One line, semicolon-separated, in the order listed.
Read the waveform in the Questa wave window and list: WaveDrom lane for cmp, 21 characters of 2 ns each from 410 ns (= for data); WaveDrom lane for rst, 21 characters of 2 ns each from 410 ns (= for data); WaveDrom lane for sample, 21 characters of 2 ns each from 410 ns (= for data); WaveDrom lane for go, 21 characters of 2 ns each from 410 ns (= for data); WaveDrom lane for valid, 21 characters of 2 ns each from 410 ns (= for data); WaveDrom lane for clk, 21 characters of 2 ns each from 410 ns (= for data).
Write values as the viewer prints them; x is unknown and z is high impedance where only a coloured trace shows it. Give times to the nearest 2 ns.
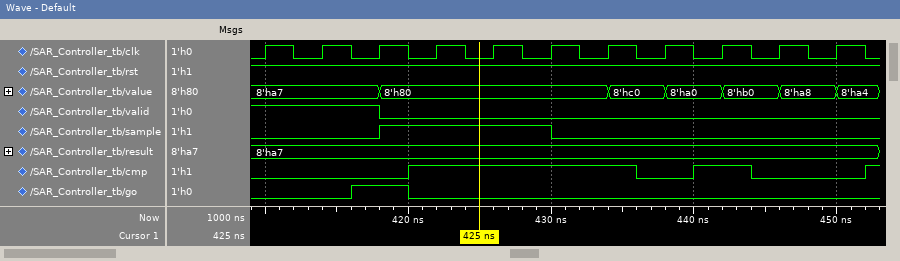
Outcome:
{name: 'cmp', wave: '0....1.......0.1.0...'}; {name: 'rst', wave: '1....................'}; {name: 'sample', wave: '0...1.....0..........'}; {name: 'go', wave: '0..1.0...............'}; {name: 'valid', wave: '1...0................'}; {name: 'clk', wave: '101010101010101010101'}
